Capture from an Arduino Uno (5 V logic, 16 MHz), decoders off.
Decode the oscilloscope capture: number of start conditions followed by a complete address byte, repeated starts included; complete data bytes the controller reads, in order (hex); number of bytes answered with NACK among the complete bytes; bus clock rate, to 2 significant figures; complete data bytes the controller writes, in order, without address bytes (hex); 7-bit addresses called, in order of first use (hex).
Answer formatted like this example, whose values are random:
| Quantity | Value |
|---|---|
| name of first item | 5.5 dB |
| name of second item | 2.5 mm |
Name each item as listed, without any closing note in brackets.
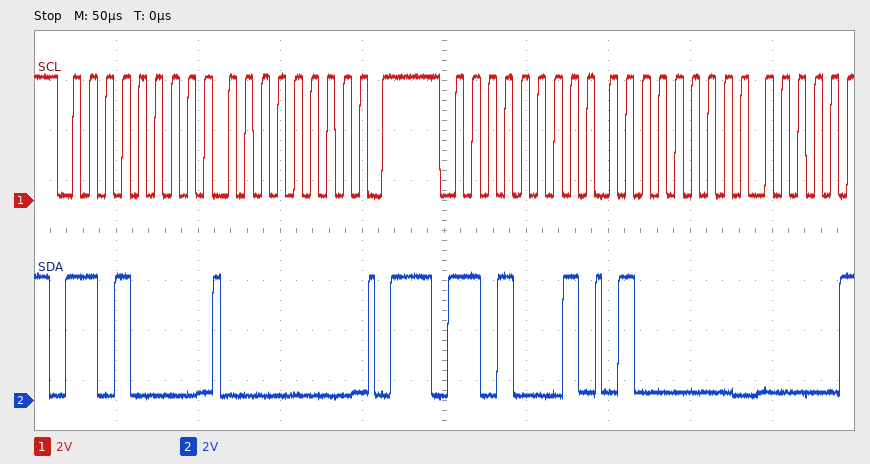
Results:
| Quantity | Value |
|---|---|
| number of start conditions followed by a complete address byte, repeated starts included | 2 |
| complete data bytes the controller reads, in order | 40 |
| number of bytes answered with NACK among the complete bytes | 0 |
| bus clock rate, to 2 significant figures | 100 kHz |
| complete data bytes the controller writes, in order, without address bytes | 00 |
| 7-bit addresses called, in order of first use | 0x68 |
